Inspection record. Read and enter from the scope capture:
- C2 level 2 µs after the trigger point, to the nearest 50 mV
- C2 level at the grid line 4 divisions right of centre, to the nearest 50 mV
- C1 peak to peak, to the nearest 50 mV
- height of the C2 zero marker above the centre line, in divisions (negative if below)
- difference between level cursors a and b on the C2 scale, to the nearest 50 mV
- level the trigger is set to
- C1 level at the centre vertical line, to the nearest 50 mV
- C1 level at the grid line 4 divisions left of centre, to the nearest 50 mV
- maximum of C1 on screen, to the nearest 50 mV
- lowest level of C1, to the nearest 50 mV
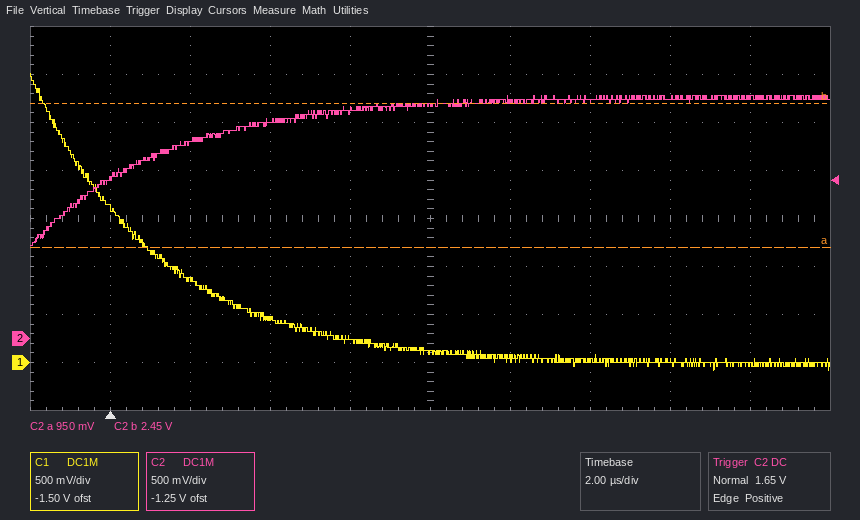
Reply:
2.05 V
2.50 V
3.10 V
-2.5 div
1.50 V
1.65 V
100 mV
1.60 V
3.00 V
-100 mV
